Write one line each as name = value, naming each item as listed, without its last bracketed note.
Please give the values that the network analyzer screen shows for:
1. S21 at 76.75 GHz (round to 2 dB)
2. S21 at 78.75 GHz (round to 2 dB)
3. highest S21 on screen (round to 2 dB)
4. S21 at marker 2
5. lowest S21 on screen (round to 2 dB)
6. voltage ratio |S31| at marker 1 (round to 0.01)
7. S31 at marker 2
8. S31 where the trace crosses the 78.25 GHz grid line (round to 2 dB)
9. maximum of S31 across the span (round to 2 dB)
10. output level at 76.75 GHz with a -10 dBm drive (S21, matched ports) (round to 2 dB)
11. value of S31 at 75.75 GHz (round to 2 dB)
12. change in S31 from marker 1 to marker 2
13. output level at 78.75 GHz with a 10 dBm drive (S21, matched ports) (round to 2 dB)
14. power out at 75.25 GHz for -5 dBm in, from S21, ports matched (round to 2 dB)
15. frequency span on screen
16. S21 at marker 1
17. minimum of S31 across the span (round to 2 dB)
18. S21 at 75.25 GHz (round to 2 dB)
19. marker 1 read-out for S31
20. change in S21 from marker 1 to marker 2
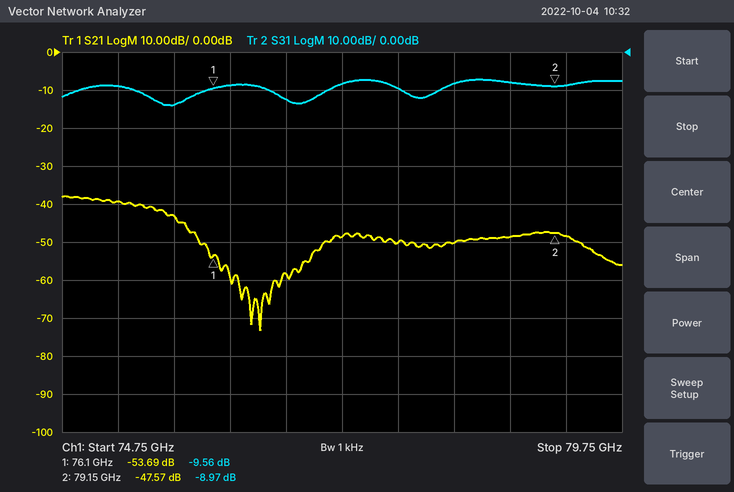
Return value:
S21 at 76.75 GHz = -58 dB
S21 at 78.75 GHz = -48 dB
highest S21 on screen = -38 dB
S21 at marker 2 = -47.57 dB
lowest S21 on screen = -74 dB
voltage ratio |S31| at marker 1 = 0.33
S31 at marker 2 = -8.97 dB
S31 where the trace crosses the 78.25 GHz grid line = -8 dB
maximum of S31 across the span = -8 dB
output level at 76.75 GHz with a -10 dBm drive (S21, matched ports) = -68 dBm
value of S31 at 75.75 GHz = -14 dB
change in S31 from marker 1 to marker 2 = 0.59 dB
output level at 78.75 GHz with a 10 dBm drive (S21, matched ports) = -38 dBm
power out at 75.25 GHz for -5 dBm in, from S21, ports matched = -44 dBm
frequency span on screen = 5 GHz
S21 at marker 1 = -53.69 dB
minimum of S31 across the span = -14 dB
S21 at 75.25 GHz = -40 dB
marker 1 read-out for S31 = -9.56 dB
change in S21 from marker 1 to marker 2 = 6.12 dB
